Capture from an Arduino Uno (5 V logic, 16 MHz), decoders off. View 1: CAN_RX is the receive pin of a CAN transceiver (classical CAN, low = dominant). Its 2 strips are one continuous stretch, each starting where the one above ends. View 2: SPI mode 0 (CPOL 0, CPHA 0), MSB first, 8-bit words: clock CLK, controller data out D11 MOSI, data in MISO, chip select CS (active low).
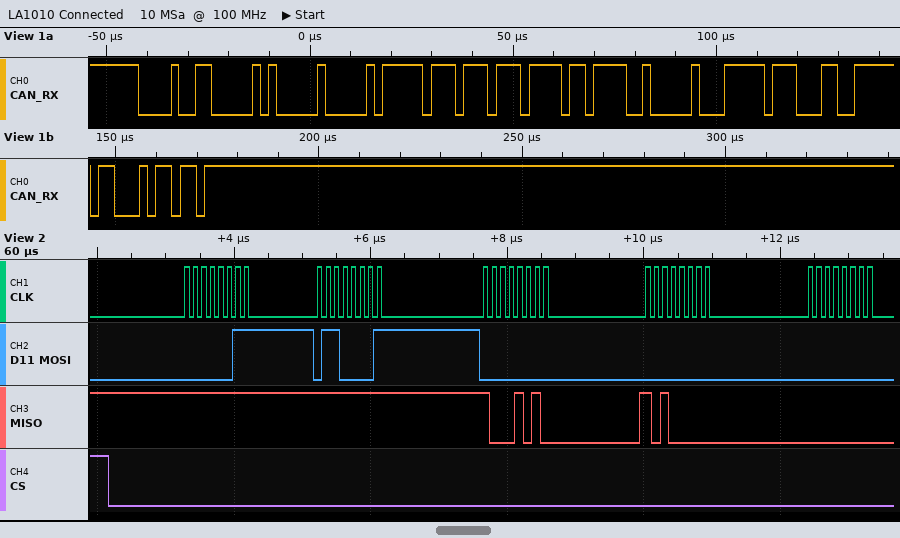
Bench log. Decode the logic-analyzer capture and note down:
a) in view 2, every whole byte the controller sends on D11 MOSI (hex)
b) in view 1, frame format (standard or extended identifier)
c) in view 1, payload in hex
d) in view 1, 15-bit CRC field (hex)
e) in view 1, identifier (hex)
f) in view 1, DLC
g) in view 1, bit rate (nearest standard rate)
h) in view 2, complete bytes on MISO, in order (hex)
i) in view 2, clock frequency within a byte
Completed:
0x03 0x61 0x00 0x00 0x00
standard
00 FF 77 7B 79 00 FF 19
0x7E2D
0x098
8
500 kbit/s
0xFF 0xFF 0x8A 0xA0 0x00
8 MHz
